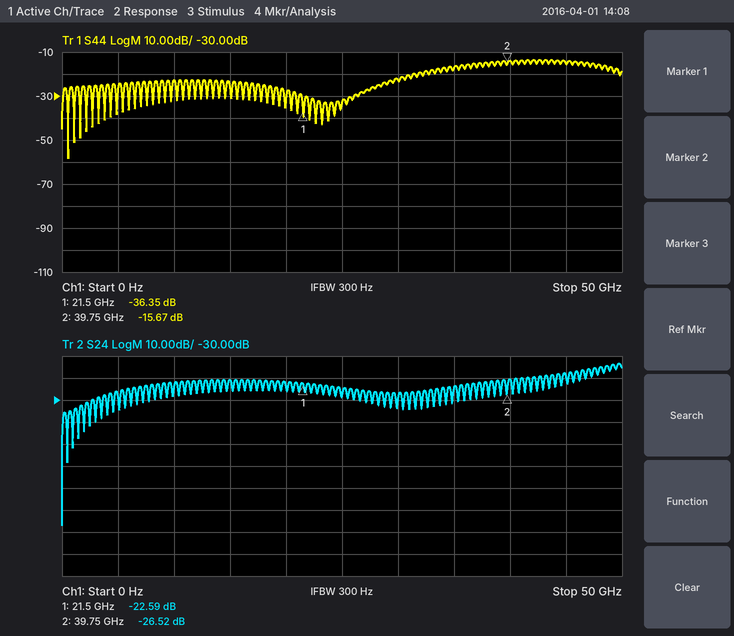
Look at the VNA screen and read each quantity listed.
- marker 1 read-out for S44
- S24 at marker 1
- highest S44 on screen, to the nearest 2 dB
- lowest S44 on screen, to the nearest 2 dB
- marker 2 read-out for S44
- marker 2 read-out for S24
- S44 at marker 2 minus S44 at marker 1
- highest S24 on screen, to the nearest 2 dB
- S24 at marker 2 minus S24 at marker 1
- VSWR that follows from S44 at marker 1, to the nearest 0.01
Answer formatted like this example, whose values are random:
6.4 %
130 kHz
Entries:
-36.35 dB
-22.59 dB
-14 dB
-58 dB
-15.67 dB
-26.52 dB
20.68 dB
-14 dB
-3.93 dB
1.03
